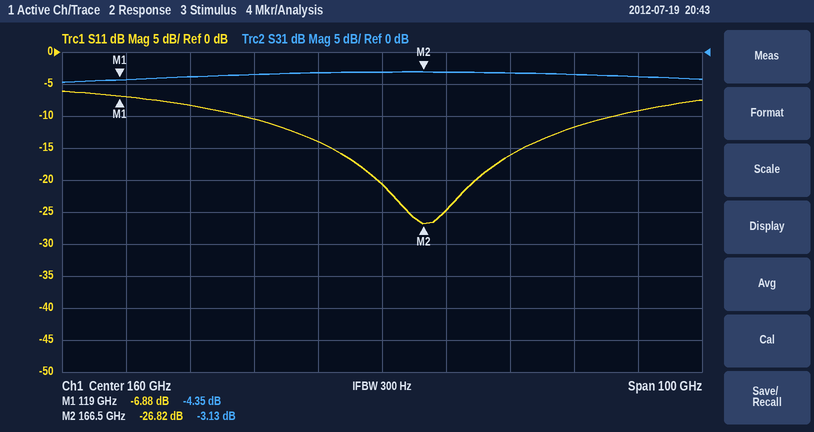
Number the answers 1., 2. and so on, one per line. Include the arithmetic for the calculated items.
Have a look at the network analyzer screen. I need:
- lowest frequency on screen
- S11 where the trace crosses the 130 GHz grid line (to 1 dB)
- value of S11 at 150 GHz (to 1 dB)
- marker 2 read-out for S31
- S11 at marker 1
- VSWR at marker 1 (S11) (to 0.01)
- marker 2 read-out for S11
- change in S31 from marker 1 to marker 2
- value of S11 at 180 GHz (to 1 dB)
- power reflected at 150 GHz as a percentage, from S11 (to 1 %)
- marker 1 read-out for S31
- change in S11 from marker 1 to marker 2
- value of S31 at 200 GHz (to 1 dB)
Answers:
1. 110 GHz
2. -8 dB
3. -14 dB
4. -3.13 dB
5. -6.88 dB
6. (1 + 0.4529)/(1 − 0.4529) ≈ 2.66
7. -26.82 dB
8. -3.13 − (-4.35) = 1.22 dB
9. -16 dB
10. 10^(-14/10) ≈ 4 %
11. -4.35 dB
12. -26.82 − (-6.88) = -19.94 dB
13. -4 dB
